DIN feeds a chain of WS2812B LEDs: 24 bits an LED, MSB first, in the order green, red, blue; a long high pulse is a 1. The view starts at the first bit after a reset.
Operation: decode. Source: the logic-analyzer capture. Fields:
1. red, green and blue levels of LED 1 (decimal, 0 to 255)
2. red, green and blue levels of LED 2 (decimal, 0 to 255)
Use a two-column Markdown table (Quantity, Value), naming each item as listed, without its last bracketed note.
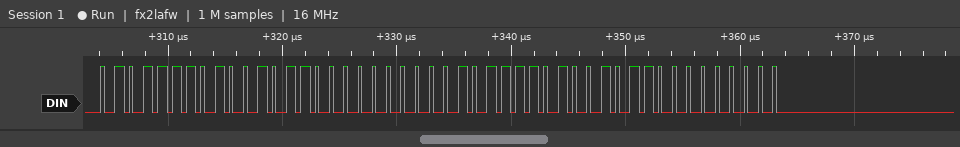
| Quantity | Value |
|---|---|
| red, green and blue levels of LED 1 | 150, 94, 0 |
| red, green and blue levels of LED 2 | 150, 94, 0 |
